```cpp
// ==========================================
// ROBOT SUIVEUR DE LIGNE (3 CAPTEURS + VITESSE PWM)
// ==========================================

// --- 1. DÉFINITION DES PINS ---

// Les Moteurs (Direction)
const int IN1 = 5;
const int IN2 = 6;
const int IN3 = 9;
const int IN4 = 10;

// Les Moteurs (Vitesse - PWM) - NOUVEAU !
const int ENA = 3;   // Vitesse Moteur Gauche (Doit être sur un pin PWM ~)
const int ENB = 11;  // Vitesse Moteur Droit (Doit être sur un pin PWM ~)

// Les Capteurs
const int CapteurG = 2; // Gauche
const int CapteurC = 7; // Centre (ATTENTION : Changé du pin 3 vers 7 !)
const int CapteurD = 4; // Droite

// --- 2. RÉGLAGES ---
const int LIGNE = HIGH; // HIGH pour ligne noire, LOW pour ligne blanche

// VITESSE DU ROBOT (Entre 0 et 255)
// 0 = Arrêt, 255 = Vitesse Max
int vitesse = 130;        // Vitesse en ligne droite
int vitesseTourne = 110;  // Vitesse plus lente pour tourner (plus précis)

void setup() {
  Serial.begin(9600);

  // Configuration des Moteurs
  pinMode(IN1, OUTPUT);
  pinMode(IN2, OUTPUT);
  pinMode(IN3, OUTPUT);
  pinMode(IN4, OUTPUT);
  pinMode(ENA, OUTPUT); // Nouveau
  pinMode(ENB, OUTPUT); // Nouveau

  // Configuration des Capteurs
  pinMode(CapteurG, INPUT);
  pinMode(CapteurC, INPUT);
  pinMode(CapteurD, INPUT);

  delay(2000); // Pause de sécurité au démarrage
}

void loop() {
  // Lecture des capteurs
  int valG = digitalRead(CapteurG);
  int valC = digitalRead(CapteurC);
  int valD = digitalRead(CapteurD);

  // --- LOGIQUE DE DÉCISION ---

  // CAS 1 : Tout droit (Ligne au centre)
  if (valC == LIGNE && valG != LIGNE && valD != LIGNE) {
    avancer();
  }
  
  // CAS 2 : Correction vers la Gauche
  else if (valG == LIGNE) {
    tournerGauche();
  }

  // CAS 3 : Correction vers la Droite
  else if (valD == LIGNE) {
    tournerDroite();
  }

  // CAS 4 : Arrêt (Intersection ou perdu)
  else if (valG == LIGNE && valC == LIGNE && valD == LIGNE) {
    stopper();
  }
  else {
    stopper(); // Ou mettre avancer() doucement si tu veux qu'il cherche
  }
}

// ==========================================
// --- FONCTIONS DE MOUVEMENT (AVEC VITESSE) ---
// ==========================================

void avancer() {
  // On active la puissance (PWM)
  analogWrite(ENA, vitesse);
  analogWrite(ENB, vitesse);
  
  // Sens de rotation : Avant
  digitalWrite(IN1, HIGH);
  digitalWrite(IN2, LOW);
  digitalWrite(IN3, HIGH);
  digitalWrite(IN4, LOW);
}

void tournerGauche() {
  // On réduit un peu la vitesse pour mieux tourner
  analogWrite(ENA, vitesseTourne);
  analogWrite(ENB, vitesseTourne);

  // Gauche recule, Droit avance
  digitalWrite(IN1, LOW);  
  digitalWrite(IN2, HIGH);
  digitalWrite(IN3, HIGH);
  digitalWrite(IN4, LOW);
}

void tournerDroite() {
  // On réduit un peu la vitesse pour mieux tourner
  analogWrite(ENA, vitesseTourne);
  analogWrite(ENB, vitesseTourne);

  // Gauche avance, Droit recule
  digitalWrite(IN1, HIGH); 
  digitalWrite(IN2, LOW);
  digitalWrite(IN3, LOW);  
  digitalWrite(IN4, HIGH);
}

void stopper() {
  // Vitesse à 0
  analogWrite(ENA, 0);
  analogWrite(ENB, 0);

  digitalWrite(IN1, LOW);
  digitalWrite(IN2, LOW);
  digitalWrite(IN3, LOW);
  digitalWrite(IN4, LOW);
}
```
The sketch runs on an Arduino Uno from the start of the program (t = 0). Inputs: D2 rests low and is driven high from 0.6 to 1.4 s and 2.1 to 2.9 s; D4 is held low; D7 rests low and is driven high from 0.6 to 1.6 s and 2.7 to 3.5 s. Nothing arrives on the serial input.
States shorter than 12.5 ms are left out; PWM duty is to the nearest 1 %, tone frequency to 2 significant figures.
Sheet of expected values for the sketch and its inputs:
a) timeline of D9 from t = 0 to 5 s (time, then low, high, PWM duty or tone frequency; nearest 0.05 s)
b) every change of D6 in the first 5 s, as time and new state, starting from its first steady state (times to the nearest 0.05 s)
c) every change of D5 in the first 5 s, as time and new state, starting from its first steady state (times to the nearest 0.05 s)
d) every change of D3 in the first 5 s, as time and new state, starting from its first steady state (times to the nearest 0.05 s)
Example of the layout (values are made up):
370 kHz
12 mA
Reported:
0 s low; 2.1 s high; 3.5 s low
0 s low; 2.1 s high; 2.9 s low
0 s low; 2.9 s high; 3.5 s low
0 s low; 2.1 s PWM 43 %; 2.9 s PWM 51 %; 3.5 s low
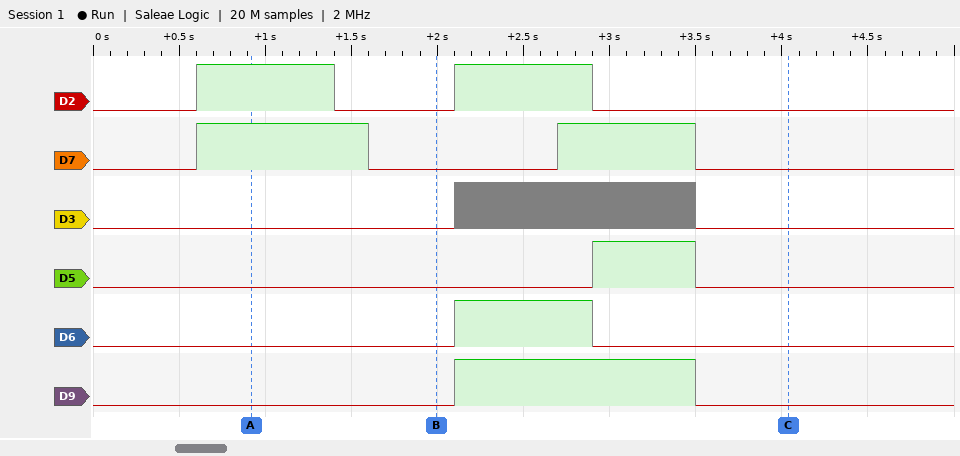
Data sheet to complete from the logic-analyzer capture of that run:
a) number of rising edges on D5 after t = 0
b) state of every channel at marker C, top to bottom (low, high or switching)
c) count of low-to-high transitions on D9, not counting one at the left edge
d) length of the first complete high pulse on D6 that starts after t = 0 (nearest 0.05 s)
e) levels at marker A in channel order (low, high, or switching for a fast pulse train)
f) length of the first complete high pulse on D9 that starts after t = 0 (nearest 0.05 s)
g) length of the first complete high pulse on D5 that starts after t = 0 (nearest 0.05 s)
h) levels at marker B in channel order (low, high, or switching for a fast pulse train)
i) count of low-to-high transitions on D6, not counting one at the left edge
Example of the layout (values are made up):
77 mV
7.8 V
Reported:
1
D2 low, D7 low, D3 low, D5 low, D6 low, D9 low
1
0.80 s
D2 high, D7 high, D3 low, D5 low, D6 low, D9 low
1.40 s
0.60 s
D2 low, D7 low, D3 low, D5 low, D6 low, D9 low
1
